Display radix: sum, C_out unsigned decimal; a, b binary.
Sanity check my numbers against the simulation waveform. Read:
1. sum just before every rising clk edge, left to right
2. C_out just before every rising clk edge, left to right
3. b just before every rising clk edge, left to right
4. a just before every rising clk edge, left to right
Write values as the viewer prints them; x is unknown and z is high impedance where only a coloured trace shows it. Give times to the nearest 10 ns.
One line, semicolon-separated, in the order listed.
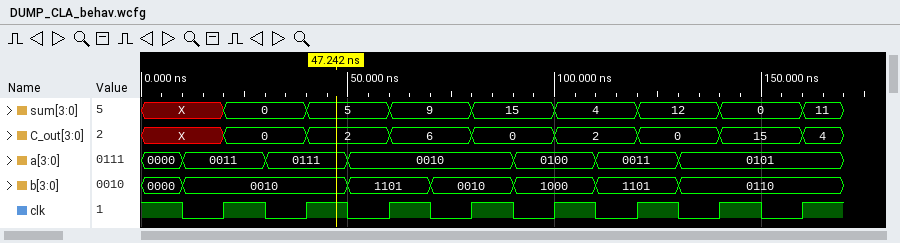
X, 0, 5, 9, 15, 4, 12, 0; X, 0, 2, 6, 0, 2, 0, 15; 0010, 0010, 1101, 0010, 1000, 1101, 0110, 0110; 0011, 0111, 0010, 0010, 0100, 0011, 0101, 0101
